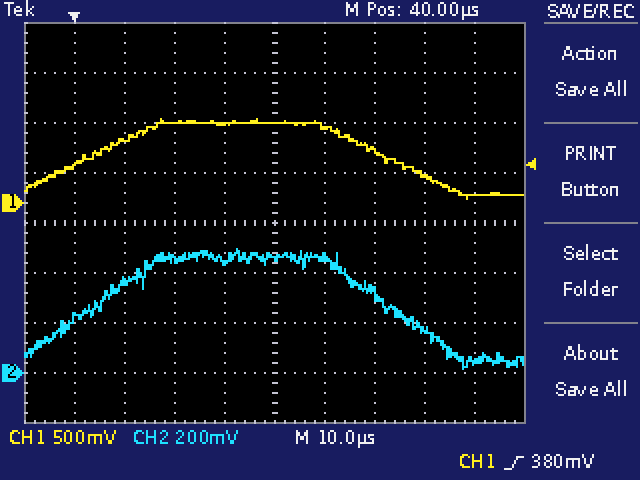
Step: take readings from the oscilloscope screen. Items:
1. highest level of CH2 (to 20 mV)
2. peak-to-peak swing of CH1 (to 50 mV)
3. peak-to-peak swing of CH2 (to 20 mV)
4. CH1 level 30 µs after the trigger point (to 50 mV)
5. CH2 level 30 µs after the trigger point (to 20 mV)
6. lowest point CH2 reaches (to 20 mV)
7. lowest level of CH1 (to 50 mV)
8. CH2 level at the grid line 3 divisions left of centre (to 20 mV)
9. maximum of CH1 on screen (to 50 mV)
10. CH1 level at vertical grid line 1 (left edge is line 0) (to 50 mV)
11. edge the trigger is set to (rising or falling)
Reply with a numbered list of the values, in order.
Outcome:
1. 500 mV
2. 800 mV
3. 480 mV
4. 800 mV
5. 440 mV
6. 20 mV
7. 50 mV
8. 360 mV
9. 850 mV
10. 400 mV
11. rising
